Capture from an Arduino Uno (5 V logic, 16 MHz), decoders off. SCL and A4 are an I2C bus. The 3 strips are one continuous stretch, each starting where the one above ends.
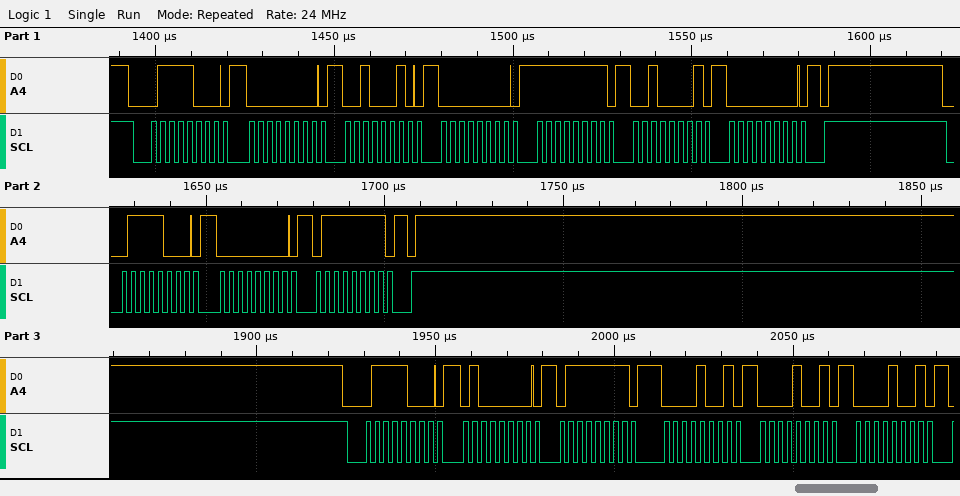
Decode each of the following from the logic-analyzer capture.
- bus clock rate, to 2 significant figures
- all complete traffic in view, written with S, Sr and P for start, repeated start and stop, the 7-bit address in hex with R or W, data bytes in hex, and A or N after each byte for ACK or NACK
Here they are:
400 kHz
S 3CW A 00 A 22 A 00 A FF A 21 A 00 A P S 3CW A 00 A 7F A P S 3CW A 40 A 7F A 09 A 09 A 09 A
